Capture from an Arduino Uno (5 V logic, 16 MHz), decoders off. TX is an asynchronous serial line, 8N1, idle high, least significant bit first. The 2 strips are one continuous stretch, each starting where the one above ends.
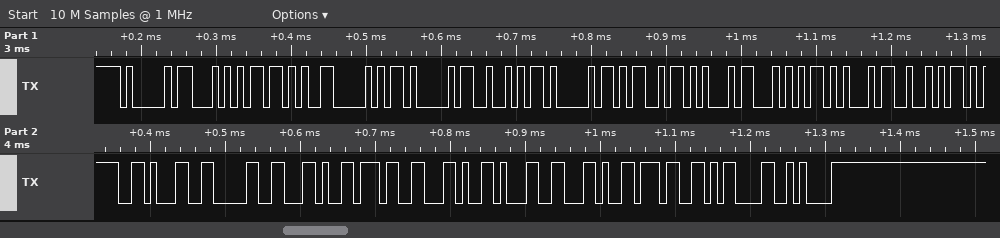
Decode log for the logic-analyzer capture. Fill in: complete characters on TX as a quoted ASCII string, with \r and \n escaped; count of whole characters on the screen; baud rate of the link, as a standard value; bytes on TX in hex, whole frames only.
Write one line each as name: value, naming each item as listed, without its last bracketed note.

complete characters on TX as a quoted ASCII string, with \r and \n escaped: "AT+PARAMETER=10,7,1,7\r\n"
count of whole characters on the screen: 23
baud rate of the link, as a standard value: 115200 baud
bytes on TX in hex, whole frames only: 41 54 2B 50 41 52 41 4D 45 54 45 52 3D 31 30 2C 37 2C 31 2C 37 0D 0A
